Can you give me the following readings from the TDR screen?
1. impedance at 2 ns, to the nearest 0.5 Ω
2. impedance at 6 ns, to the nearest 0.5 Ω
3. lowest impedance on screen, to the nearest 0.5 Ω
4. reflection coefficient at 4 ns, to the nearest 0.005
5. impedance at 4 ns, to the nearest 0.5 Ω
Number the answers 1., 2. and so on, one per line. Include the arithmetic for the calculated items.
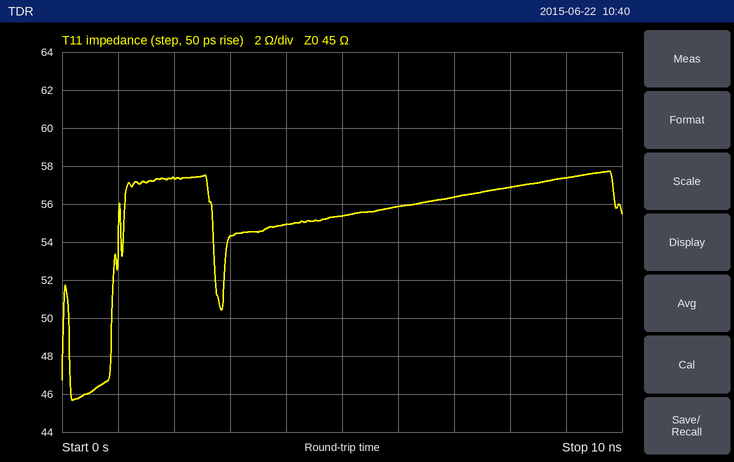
1. 57.5 Ω
2. 56.0 Ω
3. 45.5 Ω
4. (55 − 45)/(55 + 45) ≈ +0.100
5. 55.0 Ω
